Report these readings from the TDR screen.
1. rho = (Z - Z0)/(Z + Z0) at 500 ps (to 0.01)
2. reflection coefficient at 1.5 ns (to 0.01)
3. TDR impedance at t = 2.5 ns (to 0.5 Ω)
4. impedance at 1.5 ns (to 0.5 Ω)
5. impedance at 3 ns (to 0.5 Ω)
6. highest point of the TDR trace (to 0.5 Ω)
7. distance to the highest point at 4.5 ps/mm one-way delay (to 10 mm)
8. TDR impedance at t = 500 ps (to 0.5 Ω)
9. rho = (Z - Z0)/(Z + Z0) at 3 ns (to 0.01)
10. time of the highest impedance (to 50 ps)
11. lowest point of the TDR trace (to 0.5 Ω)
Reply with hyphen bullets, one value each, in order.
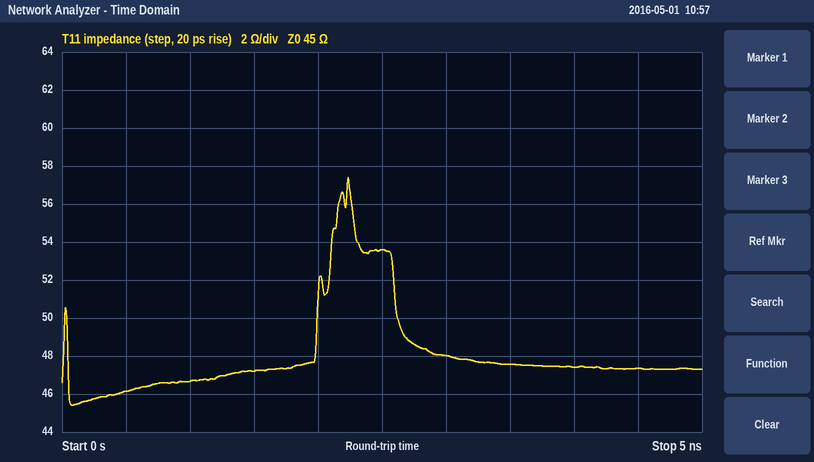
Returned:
- +0.01
- +0.02
- 53.5 Ω
- 47.0 Ω
- 48.0 Ω
- 57.5 Ω
- 250 mm
- 46.0 Ω
- +0.03
- 2.25 ns
- 45.5 Ω
